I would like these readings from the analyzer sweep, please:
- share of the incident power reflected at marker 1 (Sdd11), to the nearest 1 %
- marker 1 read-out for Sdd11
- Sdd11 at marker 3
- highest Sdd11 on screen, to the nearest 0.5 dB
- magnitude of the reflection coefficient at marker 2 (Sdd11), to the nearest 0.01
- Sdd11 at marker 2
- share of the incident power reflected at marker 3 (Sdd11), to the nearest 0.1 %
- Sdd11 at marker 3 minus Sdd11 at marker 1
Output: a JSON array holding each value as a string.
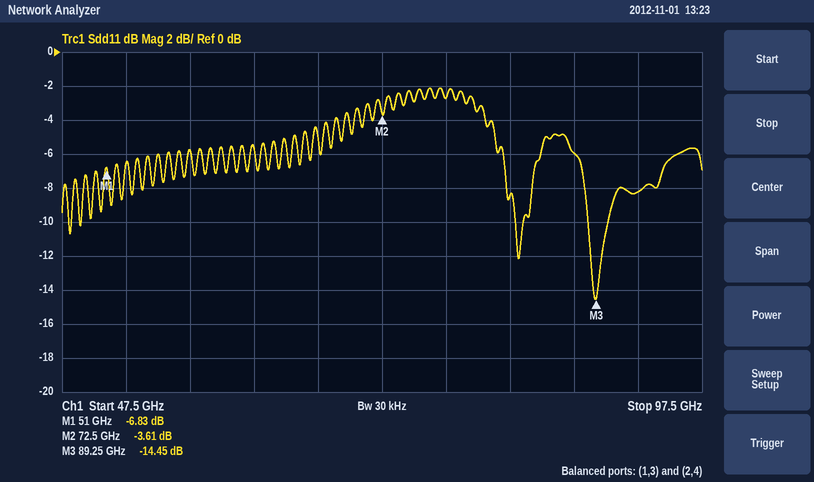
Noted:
["21 %", "-6.83 dB", "-14.45 dB", "-2.0 dB", "0.66", "-3.61 dB", "3.6 %", "-7.62 dB"]
